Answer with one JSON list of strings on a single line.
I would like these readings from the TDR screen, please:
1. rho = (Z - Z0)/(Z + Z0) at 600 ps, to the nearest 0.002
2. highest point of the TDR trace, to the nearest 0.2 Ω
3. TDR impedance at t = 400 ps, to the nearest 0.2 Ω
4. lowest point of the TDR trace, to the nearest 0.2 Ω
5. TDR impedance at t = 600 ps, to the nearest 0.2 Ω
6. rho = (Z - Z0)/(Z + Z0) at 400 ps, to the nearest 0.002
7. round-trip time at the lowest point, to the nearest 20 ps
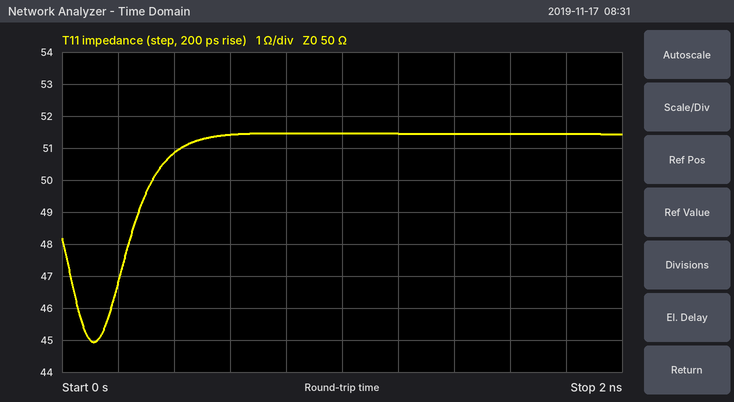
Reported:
["+0.014", "51.4 Ω", "50.8 Ω", "45.0 Ω", "51.4 Ω", "+0.008", "120 ps"]
